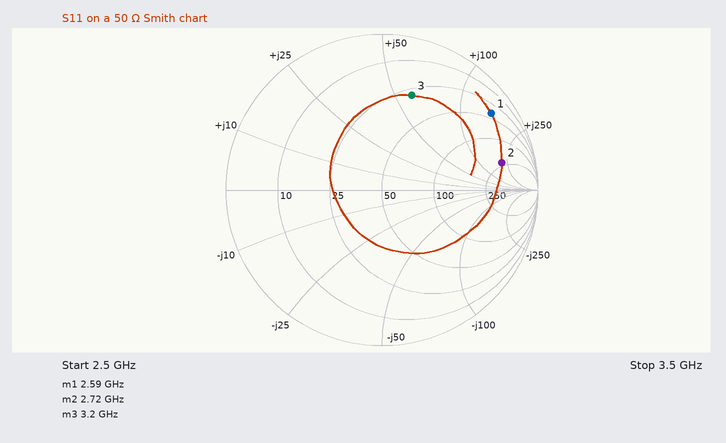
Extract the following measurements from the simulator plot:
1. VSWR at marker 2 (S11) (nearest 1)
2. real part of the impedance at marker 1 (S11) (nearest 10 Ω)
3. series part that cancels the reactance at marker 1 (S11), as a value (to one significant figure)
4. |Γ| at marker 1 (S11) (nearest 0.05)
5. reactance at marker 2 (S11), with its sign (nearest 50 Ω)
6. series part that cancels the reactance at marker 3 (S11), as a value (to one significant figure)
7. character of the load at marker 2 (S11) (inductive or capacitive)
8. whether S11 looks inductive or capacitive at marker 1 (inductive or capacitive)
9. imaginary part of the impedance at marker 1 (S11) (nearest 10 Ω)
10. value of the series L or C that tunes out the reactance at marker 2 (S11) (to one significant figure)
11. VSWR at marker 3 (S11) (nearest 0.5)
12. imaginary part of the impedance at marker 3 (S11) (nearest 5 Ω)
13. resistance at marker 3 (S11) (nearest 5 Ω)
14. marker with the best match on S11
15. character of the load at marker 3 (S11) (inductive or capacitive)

8
40 Ω
400 fF
0.85
+200 Ω
800 fF
inductive
inductive
+150 Ω
300 fF
4.5
+60 Ω
30 Ω
marker 3
inductive
